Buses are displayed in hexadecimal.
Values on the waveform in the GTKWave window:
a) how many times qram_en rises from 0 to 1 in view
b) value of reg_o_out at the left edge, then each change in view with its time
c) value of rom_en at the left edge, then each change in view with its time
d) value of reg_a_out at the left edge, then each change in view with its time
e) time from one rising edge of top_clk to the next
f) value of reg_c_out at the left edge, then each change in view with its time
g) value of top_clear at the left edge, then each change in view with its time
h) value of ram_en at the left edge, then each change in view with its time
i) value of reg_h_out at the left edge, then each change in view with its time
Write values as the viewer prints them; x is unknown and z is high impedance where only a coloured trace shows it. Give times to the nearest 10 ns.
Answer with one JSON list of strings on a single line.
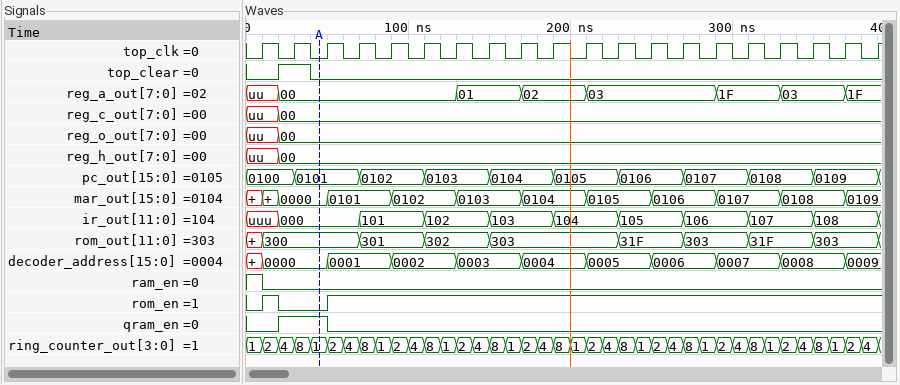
["1", "uu, 00 at 20 ns", "0, 1 at 10 ns, 0 at 20 ns, 1 at 50 ns", "uu, 00 at 20 ns, 01 at 130 ns, 02 at 170 ns, 03 at 210 ns, 1F at 290 ns, 03 at 330 ns, 1F at 370 ns", "20 ns", "uu, 00 at 20 ns", "0, 1 at 20 ns, 0 at 40 ns", "1, 0 at 10 ns", "uu, 00 at 20 ns"]
